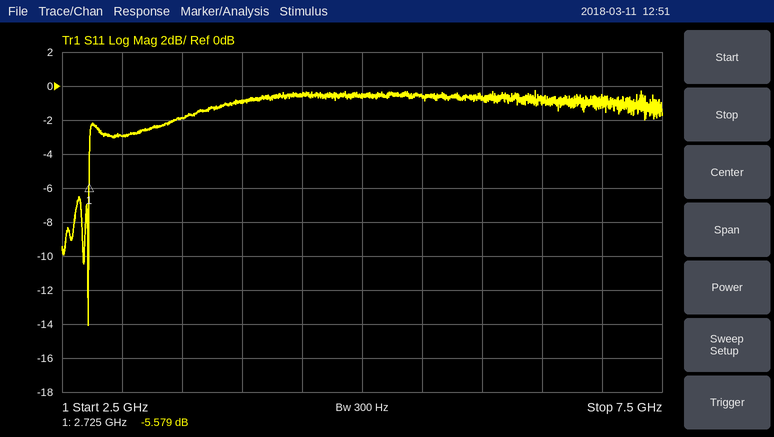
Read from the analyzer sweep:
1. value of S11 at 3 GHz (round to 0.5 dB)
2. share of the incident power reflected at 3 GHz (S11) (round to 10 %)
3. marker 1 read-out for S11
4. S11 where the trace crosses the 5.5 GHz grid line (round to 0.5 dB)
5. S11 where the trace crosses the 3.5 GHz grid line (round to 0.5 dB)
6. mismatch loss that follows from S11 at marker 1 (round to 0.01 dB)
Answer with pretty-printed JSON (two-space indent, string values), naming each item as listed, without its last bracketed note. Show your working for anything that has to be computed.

{
  "value of S11 at 3 GHz": "-3.0 dB",
  "share of the incident power reflected at 3 GHz (S11)": "10^(-3/10) ≈ 50 %",
  "marker 1 read-out for S11": "-5.579 dB",
  "S11 where the trace crosses the 5.5 GHz grid line": "-0.5 dB",
  "S11 where the trace crosses the 3.5 GHz grid line": "-2.0 dB",
  "mismatch loss that follows from S11 at marker 1": "−10 log10(1 − 10^(-5.579/10)) ≈ 1.41 dB"
}
